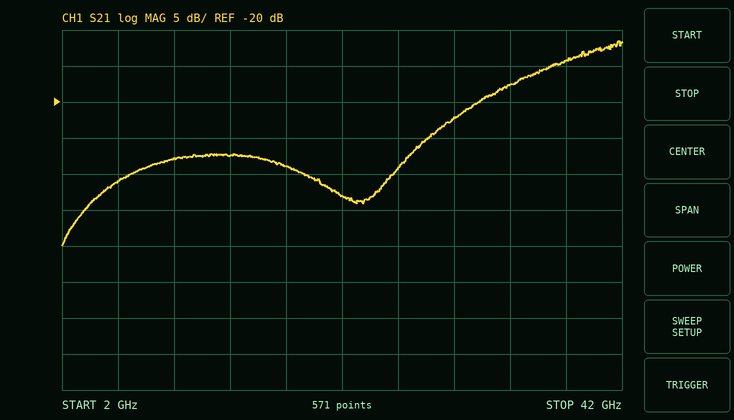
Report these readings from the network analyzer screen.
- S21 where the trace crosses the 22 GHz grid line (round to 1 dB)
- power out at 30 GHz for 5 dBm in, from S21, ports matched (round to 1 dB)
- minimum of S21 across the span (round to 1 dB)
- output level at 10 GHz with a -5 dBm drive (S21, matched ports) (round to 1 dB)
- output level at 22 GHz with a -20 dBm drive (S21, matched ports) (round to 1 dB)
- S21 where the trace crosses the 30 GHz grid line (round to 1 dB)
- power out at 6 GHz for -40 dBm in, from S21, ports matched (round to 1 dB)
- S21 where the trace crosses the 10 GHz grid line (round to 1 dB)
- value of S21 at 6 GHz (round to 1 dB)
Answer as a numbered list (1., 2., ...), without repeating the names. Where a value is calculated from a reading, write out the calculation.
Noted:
1. -33 dB
2. 5 dBm + (-22 dB) = -17 dBm
3. -40 dB
4. -5 dBm + (-28 dB) = -33 dBm
5. -20 dBm + (-33 dB) = -53 dBm
6. -22 dB
7. -40 dBm + (-31 dB) = -71 dBm
8. -28 dB
9. -31 dB
